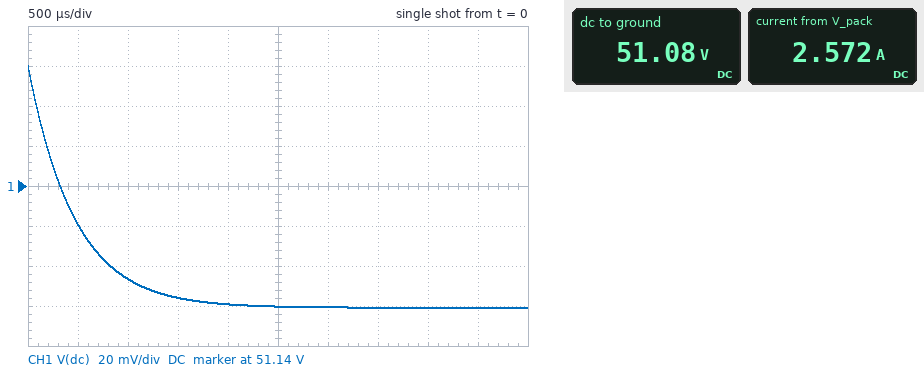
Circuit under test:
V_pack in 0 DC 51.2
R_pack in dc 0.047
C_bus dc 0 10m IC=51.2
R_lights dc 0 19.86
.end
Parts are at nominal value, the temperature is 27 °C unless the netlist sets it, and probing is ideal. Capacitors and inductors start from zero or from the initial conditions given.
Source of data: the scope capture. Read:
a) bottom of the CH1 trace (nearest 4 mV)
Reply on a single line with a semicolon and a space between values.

51.080 V
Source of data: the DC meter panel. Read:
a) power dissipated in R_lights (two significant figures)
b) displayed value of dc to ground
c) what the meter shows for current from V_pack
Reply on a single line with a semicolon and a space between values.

130 W; 51.08 V; 2.572 A
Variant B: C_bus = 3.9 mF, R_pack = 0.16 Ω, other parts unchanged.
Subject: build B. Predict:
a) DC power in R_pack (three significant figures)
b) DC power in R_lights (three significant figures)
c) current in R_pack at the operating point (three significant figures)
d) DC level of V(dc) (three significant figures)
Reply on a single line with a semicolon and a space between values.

1.05 W; 130 W; 2.56 A; 50.8 V
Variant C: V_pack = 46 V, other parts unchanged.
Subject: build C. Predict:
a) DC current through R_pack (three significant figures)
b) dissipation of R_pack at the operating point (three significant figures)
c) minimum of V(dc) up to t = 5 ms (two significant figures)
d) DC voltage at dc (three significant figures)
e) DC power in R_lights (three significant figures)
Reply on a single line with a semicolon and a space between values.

2.31 A; 251 mW; 46 V; 45.9 V; 106 W
